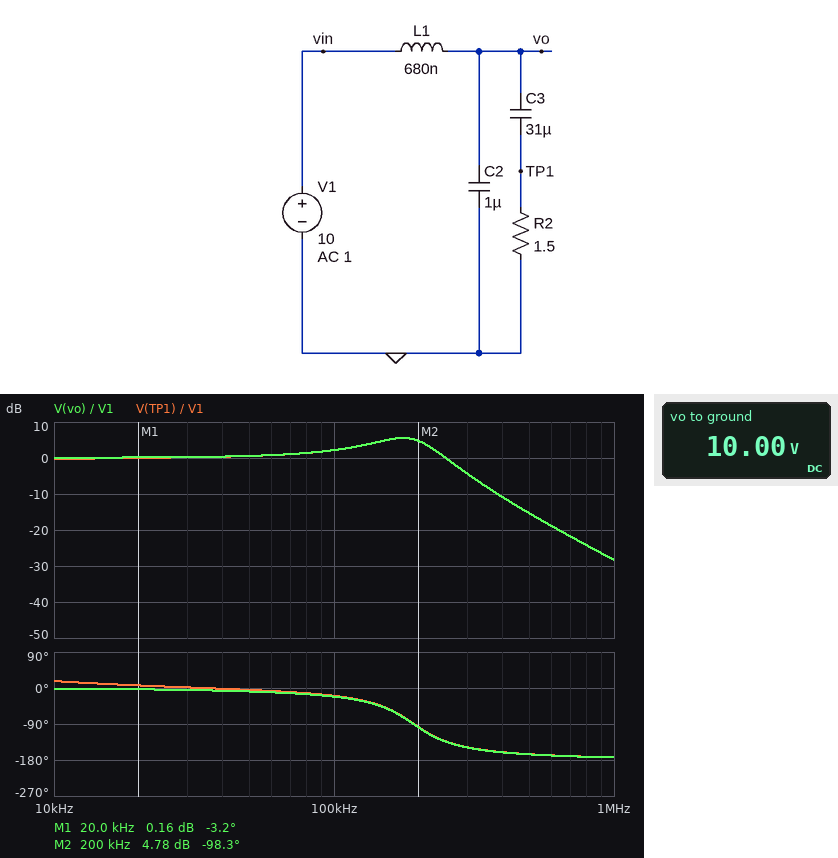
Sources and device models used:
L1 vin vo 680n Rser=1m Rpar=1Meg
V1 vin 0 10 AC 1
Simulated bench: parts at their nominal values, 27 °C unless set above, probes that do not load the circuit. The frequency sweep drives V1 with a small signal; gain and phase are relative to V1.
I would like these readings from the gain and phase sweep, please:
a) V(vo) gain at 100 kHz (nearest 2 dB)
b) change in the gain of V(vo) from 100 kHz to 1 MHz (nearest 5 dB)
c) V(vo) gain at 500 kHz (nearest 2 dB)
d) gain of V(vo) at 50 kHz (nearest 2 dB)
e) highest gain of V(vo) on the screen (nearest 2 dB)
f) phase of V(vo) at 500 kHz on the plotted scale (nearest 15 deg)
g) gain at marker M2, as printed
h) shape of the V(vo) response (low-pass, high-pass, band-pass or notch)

2 dB
-30 dB
-16 dB
0 dB
6 dB
-165 deg
4.78 dB
low-pass
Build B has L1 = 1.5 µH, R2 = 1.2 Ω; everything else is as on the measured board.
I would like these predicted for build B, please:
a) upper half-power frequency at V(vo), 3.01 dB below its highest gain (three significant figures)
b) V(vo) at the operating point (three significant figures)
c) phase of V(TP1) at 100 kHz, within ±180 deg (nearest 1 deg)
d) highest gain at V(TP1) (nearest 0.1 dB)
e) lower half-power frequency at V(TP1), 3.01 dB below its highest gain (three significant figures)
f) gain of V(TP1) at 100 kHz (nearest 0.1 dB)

148 kHz
10.0 V
-62 deg
1.3 dB
5.81 kHz
1.2 dB
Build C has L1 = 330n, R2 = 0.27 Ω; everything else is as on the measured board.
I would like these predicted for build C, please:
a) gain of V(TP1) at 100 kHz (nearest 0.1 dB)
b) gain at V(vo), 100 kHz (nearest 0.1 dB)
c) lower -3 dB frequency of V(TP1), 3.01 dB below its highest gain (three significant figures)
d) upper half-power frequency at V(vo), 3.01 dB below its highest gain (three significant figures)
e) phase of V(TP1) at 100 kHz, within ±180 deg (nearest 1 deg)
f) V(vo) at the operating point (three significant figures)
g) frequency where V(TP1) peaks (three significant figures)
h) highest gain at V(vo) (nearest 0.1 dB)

-0.5 dB
-0.4 dB
17.7 kHz
150 kHz
-35 deg
10.0 V
55.6 kHz
0.9 dB
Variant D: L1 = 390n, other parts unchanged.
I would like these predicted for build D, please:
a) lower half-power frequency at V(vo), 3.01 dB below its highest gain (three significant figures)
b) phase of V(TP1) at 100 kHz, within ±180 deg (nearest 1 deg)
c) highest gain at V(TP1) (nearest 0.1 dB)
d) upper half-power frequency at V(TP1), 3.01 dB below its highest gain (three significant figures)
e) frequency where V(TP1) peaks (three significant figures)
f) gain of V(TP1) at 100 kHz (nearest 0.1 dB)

180 kHz
-9 deg
7.8 dB
292 kHz
243 kHz
1.3 dB
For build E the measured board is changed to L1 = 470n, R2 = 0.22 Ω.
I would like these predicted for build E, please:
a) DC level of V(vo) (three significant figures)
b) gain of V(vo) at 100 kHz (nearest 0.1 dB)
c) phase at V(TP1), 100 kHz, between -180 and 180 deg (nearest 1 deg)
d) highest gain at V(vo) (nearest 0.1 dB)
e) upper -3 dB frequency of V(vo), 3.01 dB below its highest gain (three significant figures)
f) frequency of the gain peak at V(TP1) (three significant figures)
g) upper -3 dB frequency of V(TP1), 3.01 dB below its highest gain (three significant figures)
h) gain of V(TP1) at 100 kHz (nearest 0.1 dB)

10.0 V
-2.8 dB
-55 deg
1.6 dB
81.5 kHz
43.2 kHz
96.4 kHz
-3.0 dB
